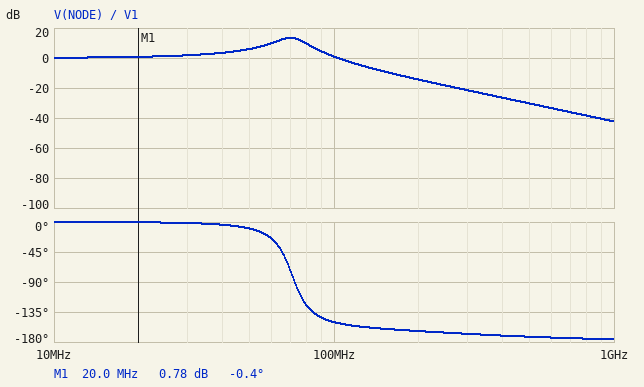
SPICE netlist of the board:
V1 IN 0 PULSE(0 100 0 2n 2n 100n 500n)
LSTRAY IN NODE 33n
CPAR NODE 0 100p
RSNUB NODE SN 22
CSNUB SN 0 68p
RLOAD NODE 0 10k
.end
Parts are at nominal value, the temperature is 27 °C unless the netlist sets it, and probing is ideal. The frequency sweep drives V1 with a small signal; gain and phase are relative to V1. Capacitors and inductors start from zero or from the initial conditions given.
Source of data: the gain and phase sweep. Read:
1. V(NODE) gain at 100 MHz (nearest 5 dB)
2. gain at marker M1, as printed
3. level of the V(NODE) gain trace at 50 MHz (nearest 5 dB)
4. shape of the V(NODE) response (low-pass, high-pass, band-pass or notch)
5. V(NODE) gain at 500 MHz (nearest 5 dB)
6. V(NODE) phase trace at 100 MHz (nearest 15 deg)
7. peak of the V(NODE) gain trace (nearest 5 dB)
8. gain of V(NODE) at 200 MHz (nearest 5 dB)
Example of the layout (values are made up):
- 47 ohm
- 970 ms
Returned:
- 0 dB
- 0.78 dB
- 5 dB
- low-pass
- -30 dB
- -150 deg
- 15 dB
- -15 dB
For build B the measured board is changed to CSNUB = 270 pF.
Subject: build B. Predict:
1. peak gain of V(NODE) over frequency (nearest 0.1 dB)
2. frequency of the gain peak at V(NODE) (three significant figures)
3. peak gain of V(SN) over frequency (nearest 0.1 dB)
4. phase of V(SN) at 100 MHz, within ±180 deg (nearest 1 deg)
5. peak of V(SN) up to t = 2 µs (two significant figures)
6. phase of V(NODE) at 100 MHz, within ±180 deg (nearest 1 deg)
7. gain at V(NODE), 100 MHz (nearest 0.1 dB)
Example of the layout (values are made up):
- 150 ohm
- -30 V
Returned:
- 4.9 dB
- 61.3 MHz
- 0 dB
- 164 deg
- 100 V
- -121 deg
- -0.3 dB
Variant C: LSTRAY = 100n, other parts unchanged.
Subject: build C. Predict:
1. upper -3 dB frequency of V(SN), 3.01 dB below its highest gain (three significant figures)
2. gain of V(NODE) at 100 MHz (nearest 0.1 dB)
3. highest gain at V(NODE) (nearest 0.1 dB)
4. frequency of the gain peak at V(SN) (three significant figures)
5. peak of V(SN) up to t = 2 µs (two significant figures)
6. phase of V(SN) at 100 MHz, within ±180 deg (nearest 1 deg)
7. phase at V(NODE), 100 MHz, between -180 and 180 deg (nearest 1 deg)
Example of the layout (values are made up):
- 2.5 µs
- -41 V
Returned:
- 42.0 MHz
- -13.2 dB
- 17.1 dB
- 39.2 MHz
- 180 V
- 154 deg
- -163 deg
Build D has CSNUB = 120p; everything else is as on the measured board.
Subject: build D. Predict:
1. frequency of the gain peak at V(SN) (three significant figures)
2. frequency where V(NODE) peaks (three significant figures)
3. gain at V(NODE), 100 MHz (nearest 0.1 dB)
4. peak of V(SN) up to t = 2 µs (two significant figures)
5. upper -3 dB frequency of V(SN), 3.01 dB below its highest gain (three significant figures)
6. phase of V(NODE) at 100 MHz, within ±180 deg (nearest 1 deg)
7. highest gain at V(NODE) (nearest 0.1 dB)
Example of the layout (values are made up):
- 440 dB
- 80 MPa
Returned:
- 62.6 MHz
- 64.7 MHz
- 0 dB
- 140 V
- 76.4 MHz
- -136 deg
- 8.9 dB
